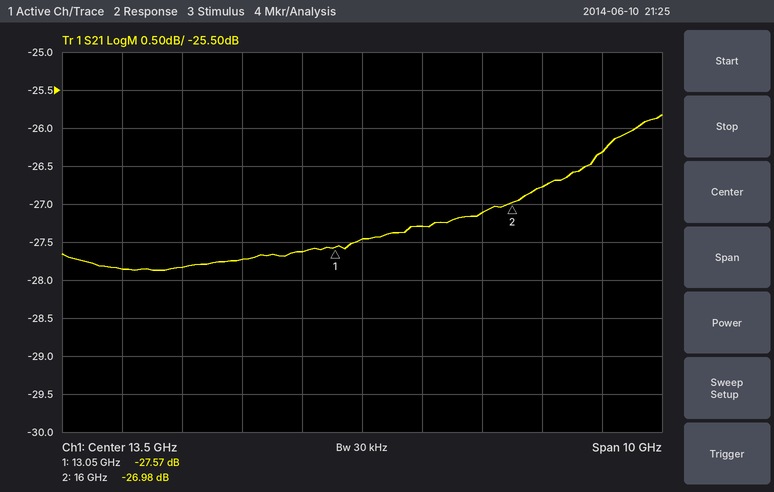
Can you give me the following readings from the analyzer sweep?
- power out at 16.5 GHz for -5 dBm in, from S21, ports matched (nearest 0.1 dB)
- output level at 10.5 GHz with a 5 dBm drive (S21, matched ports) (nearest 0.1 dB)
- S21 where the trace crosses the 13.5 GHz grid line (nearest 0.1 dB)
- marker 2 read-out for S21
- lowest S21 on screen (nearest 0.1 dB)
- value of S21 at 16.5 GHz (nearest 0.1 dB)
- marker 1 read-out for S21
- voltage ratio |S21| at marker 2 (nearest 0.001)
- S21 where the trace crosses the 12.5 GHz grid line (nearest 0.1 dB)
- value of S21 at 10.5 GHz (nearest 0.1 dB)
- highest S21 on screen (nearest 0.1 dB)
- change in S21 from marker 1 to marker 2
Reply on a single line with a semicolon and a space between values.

-31.8 dBm; -22.8 dBm; -27.5 dB; -26.98 dB; -27.9 dB; -26.8 dB; -27.57 dB; 0.045; -27.6 dB; -27.8 dB; -25.8 dB; 0.59 dB
